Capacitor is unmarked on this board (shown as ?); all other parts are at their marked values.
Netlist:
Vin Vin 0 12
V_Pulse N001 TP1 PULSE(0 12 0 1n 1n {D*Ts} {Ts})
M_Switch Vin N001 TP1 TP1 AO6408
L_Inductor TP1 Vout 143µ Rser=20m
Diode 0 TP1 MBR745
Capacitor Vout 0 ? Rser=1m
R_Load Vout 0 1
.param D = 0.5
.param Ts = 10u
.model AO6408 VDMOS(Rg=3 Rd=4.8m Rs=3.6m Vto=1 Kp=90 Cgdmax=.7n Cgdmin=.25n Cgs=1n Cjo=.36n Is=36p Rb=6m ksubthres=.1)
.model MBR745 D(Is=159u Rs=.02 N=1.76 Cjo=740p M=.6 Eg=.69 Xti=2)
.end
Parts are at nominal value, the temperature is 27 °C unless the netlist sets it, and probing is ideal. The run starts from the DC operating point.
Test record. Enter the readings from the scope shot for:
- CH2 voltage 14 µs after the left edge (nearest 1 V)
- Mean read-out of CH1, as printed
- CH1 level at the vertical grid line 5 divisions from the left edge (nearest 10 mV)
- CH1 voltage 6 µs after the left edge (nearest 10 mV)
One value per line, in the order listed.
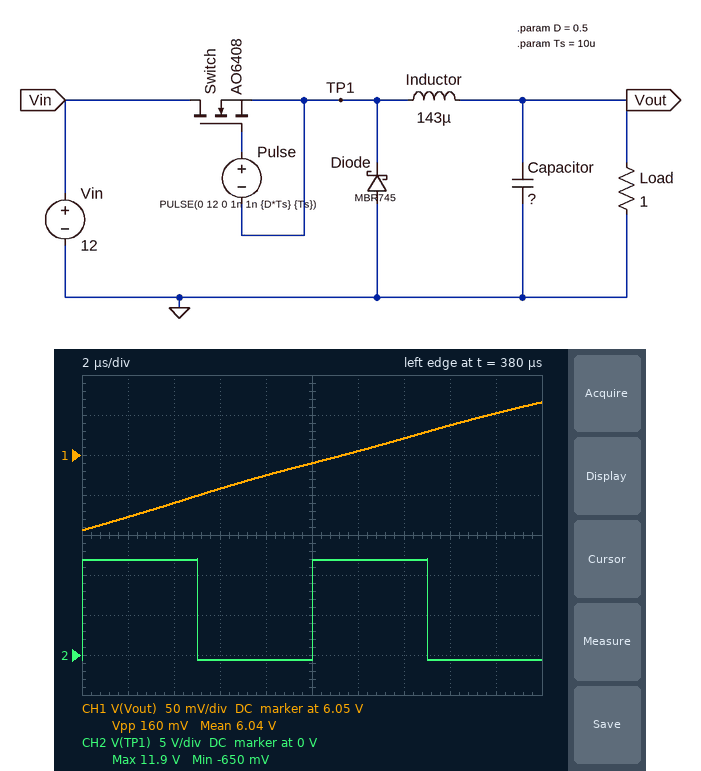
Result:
12 V
6.04 V
6.04 V
6.01 V
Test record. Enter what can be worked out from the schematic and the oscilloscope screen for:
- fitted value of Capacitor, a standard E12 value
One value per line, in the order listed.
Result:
150 µF
